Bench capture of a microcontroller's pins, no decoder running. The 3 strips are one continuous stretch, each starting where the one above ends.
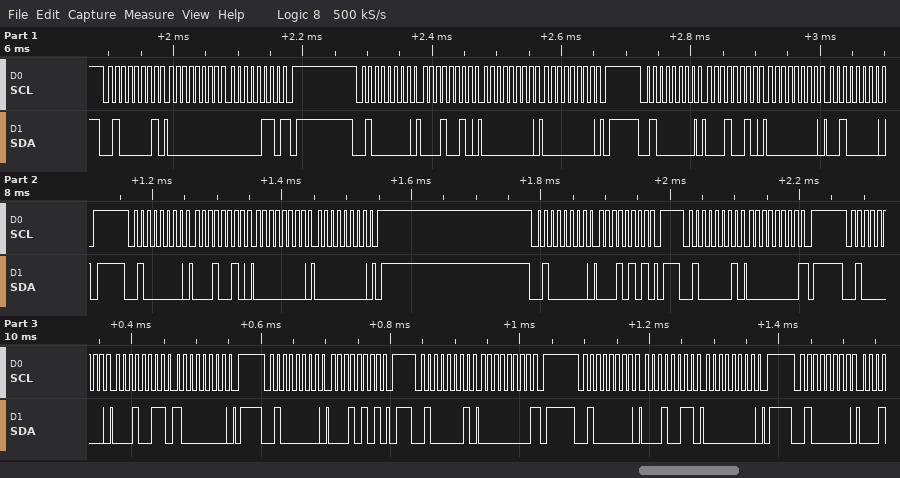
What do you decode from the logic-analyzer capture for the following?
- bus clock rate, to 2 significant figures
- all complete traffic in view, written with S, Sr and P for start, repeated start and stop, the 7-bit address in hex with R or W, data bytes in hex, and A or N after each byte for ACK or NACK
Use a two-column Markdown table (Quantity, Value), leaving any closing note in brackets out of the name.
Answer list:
| Quantity | Value |
|---|---|
| bus clock rate, to 2 significant figures | 100 kHz |
| all complete traffic in view, written with S, Sr and P for start, repeated start and stop, the 7-bit address in hex with R or W, data bytes in hex, and A or N after each byte for ACK or NACK | S 20R A 00 A 06 N P S 20W A 12 A 00 A 00 A P S 20W A 12 A 00 A 20 A P S 20W A 12 A 00 A 00 A P S 20W A 15 A P S 20R A 00 N P S 20W A 13 A 80 A P S 20W A 15 A P S 20R A 00 N P S 20W A 13 A 00 A P S 20W A |
